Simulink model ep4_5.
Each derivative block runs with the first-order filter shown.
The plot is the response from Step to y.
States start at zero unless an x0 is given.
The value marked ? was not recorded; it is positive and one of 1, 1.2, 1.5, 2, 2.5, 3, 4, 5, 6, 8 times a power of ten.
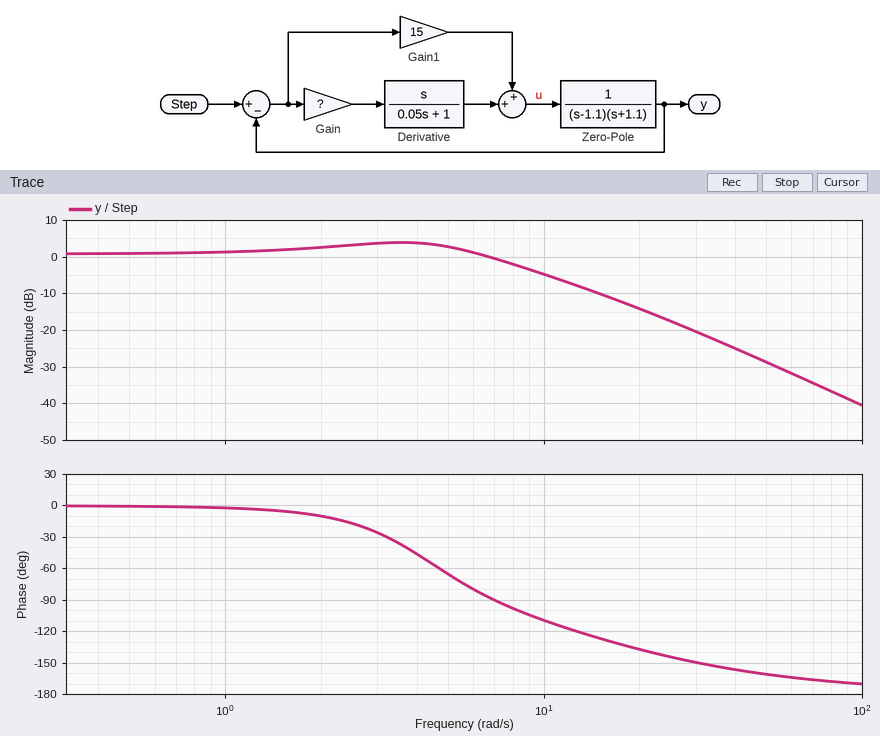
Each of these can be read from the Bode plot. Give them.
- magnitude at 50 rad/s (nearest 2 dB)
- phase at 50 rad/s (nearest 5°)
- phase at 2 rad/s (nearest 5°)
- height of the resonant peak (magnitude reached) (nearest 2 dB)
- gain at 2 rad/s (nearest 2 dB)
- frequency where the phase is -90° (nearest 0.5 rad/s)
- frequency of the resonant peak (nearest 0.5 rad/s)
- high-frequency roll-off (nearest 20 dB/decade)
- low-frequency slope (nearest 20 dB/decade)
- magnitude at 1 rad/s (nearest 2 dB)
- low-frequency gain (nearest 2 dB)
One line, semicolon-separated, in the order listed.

-28 dB; -160°; -10°; 4 dB; 2 dB; 7.0 rad/s; 3.5 rad/s; -40 dB/decade; 0 dB/decade; 2 dB; 0 dB
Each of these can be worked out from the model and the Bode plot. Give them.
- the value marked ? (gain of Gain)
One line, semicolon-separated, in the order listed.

4
